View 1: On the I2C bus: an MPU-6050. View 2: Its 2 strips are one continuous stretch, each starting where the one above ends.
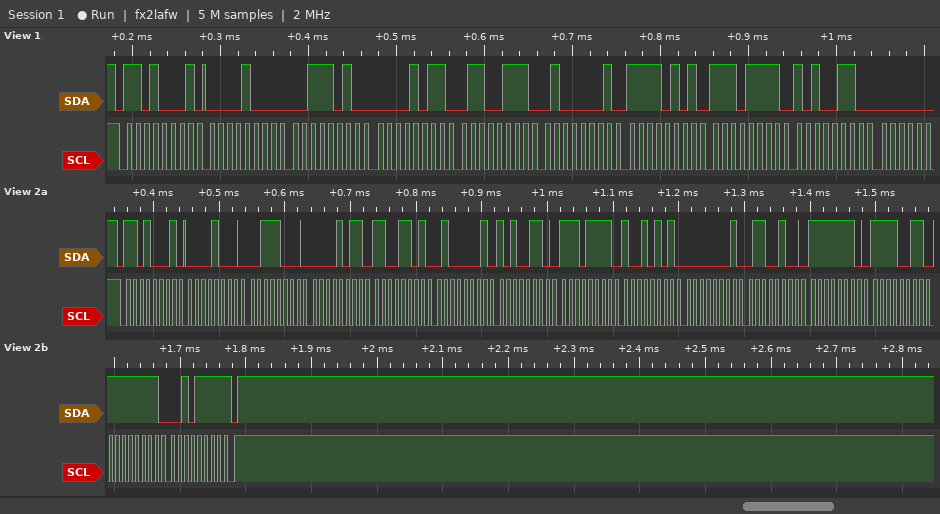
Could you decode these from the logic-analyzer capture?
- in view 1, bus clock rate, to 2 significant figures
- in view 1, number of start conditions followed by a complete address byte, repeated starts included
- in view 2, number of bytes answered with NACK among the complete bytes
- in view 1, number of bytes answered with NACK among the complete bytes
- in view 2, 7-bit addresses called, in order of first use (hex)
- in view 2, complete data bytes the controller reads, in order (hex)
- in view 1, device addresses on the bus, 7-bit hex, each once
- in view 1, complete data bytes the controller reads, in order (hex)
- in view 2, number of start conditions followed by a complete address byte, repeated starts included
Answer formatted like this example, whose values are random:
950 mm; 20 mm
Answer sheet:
100 kHz; 1; 1; 0; 0x68; 08 38 0B CD 41 A6 EF 95 01 64 FE F3 FF 2F; 0x68; 08 3A 0B 67 41 F5 EF A6; 1
